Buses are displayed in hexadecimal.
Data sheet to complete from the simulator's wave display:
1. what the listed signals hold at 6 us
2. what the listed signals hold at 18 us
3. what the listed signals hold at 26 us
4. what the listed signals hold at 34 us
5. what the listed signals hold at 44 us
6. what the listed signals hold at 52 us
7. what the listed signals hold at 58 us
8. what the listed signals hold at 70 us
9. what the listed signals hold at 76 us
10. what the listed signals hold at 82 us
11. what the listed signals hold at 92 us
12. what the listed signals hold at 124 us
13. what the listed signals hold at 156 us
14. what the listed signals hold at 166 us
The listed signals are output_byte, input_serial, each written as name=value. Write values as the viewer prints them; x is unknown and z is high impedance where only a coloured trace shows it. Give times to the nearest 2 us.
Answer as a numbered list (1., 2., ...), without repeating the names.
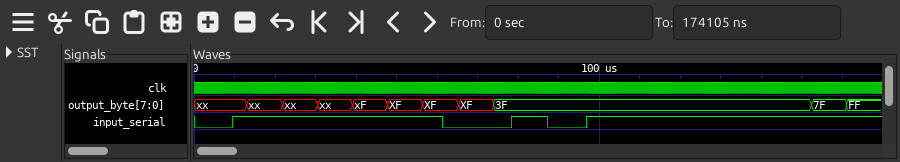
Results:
1. output_byte=xx, input_serial=0
2. output_byte=xx, input_serial=1
3. output_byte=xx, input_serial=1
4. output_byte=xx, input_serial=1
5. output_byte=xF, input_serial=1
6. output_byte=XF, input_serial=1
7. output_byte=XF, input_serial=1
8. output_byte=XF, input_serial=0
9. output_byte=3F, input_serial=0
10. output_byte=3F, input_serial=1
11. output_byte=3F, input_serial=0
12. output_byte=3F, input_serial=1
13. output_byte=7F, input_serial=1
14. output_byte=FF, input_serial=1
